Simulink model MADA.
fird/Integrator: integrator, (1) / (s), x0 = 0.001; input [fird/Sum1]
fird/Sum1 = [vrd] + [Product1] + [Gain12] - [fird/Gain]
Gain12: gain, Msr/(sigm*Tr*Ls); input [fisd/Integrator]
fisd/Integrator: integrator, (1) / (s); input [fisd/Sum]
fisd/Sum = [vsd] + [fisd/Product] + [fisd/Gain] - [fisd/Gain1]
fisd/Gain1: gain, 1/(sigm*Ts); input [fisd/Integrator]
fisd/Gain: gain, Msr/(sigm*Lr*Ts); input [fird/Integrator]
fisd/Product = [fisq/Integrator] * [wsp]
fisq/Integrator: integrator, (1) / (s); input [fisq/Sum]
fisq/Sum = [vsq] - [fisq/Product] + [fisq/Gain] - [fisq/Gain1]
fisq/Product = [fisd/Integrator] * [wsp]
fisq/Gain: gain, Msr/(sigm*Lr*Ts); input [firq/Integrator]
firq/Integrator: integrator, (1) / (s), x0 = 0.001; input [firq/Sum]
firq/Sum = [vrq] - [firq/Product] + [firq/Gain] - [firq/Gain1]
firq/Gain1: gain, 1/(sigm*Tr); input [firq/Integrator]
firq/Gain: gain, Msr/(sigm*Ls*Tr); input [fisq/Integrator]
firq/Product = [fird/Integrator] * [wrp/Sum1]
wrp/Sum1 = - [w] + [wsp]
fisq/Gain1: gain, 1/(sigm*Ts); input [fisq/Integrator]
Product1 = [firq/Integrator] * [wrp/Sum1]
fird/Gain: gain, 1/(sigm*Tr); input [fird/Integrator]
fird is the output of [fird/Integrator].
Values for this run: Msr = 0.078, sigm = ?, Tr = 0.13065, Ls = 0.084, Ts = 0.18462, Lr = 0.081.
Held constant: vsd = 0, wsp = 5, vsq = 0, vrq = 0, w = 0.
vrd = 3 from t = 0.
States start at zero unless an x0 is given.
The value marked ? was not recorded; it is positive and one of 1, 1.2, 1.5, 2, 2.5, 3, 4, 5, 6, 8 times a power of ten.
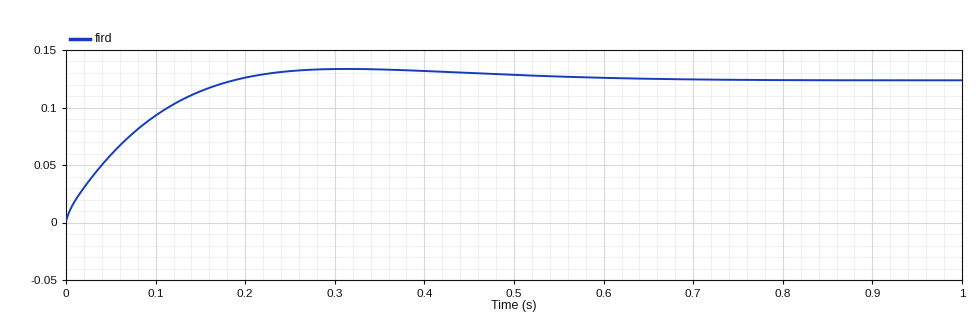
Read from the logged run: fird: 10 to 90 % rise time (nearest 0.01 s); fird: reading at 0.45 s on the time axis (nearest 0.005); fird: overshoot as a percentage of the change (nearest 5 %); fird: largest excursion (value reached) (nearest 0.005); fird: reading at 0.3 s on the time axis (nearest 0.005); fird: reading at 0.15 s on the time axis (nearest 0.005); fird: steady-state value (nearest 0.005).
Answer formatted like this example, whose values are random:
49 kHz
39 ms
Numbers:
0.14 s
0.130
10 %
0.135
0.135
0.115
0.125
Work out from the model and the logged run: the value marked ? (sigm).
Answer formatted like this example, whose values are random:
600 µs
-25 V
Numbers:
0.05
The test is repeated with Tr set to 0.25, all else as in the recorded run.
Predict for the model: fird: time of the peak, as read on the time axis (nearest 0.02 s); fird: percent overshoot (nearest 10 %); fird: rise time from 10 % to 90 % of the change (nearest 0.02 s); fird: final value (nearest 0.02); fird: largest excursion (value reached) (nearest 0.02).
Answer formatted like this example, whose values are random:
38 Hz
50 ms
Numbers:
0.32 s
20 %
0.12 s
0.18
0.22
